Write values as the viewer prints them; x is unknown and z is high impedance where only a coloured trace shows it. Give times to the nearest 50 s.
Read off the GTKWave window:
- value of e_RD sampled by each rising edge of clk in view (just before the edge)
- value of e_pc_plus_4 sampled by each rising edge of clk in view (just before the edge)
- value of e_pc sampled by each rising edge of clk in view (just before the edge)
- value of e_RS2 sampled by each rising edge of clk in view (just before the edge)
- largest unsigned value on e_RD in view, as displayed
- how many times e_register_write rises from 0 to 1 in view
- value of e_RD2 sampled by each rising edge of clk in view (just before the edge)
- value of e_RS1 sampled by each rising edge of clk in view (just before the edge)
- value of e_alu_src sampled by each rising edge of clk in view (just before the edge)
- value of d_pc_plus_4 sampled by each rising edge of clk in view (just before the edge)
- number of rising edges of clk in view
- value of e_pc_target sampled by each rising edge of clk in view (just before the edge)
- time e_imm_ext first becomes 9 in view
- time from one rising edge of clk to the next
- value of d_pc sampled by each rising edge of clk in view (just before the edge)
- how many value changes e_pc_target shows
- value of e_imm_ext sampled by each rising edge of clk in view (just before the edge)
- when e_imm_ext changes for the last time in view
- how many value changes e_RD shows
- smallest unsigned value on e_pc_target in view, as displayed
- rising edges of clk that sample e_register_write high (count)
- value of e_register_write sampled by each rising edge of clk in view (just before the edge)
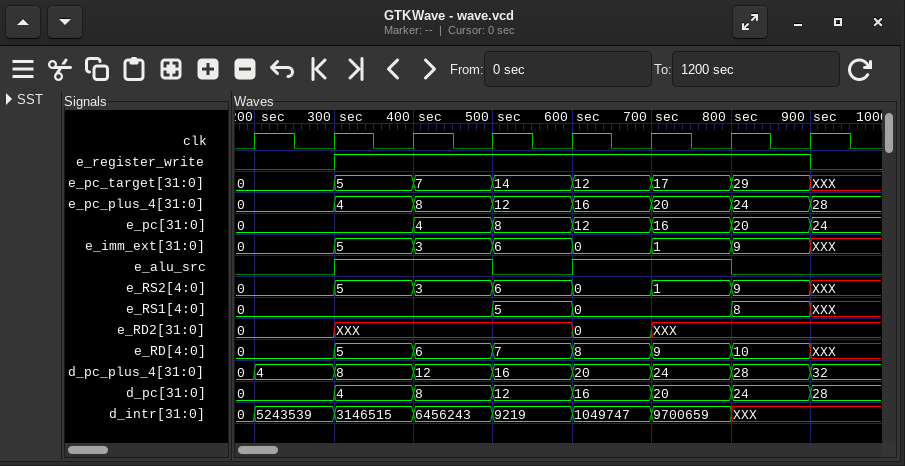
0, 0, 5, 6, 7, 8, 9, 10
0, 0, 4, 8, 12, 16, 20, 24
0, 0, 0, 4, 8, 12, 16, 20
0, 0, 5, 3, 6, 0, 1, 9
10
1
0, 0, XXX, XXX, XXX, 0, XXX, XXX
0, 0, 0, 0, 5, 0, 0, 8
0 0 1 1 0 1 1 0
0, 4, 8, 12, 16, 20, 24, 28
8
0, 0, 5, 7, 14, 12, 17, 29
800 s
100 s
0, 0, 4, 8, 12, 16, 20, 24
7
0, 0, 5, 3, 6, 0, 1, 9
900 s
7
0
6
0 0 1 1 1 1 1 1
